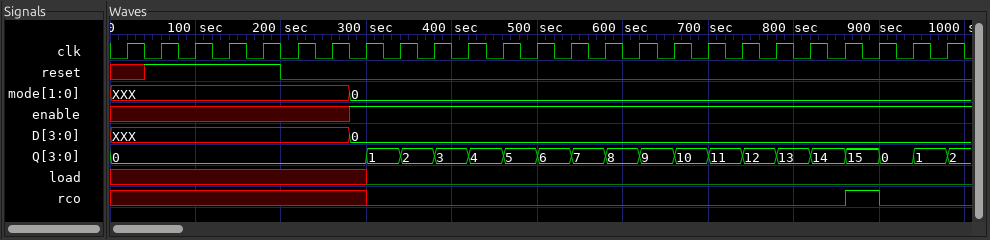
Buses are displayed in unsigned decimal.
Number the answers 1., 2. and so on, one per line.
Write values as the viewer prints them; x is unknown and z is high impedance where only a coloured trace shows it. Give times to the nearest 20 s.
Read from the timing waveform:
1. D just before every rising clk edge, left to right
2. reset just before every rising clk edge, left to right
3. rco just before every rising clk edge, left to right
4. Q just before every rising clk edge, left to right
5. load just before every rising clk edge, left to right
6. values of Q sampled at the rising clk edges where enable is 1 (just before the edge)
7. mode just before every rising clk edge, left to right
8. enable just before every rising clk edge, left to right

1. XXX, XXX, XXX, XXX, XXX, XXX, XXX, 0, 0, 0, 0, 0, 0, 0, 0, 0, 0, 0, 0, 0, 0, 0, 0, 0, 0
2. x 1 1 1 1 0 0 0 0 0 0 0 0 0 0 0 0 0 0 0 0 0 0 0 0
3. x x x x x x x x 0 0 0 0 0 0 0 0 0 0 0 0 0 0 1 0 0
4. 0, 0, 0, 0, 0, 0, 0, 0, 1, 2, 3, 4, 5, 6, 7, 8, 9, 10, 11, 12, 13, 14, 15, 0, 1
5. x x x x x x x x 0 0 0 0 0 0 0 0 0 0 0 0 0 0 0 0 0
6. 0, 1, 2, 3, 4, 5, 6, 7, 8, 9, 10, 11, 12, 13, 14, 15, 0, 1
7. XXX, XXX, XXX, XXX, XXX, XXX, XXX, 0, 0, 0, 0, 0, 0, 0, 0, 0, 0, 0, 0, 0, 0, 0, 0, 0, 0
8. x x x x x x x 1 1 1 1 1 1 1 1 1 1 1 1 1 1 1 1 1 1
